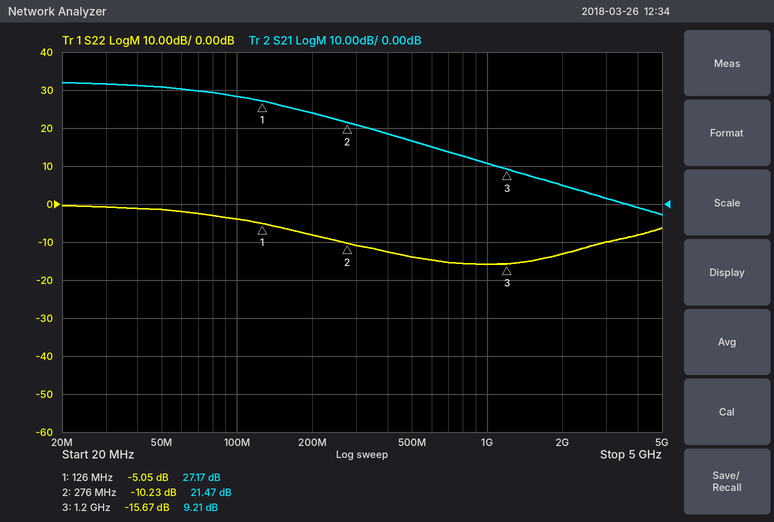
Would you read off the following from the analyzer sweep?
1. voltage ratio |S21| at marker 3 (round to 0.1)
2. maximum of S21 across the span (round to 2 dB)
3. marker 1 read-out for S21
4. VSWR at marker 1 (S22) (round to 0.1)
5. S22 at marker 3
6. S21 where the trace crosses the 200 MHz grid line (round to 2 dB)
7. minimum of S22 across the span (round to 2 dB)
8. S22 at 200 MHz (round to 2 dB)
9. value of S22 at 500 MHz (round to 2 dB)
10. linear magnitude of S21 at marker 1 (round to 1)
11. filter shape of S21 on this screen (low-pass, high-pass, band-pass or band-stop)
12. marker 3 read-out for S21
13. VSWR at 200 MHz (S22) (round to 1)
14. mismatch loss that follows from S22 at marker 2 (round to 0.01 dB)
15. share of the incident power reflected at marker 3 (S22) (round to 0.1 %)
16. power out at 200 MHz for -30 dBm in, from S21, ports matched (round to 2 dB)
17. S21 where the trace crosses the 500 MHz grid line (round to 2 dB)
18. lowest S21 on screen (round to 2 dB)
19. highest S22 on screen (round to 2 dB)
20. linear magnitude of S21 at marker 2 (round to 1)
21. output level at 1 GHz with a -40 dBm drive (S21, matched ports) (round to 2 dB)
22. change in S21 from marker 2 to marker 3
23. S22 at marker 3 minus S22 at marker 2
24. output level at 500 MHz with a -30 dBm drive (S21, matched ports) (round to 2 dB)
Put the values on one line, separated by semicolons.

2.9; 32 dB; 27.17 dB; 3.5; -15.67 dB; 24 dB; -16 dB; -8 dB; -14 dB; 23; low-pass; 9.21 dB; 2; 0.43 dB; 2.7 %; -6 dBm; 16 dB; -2 dB; 0 dB; 12; -30 dBm; -12.26 dB; -5.44 dB; -14 dBm
